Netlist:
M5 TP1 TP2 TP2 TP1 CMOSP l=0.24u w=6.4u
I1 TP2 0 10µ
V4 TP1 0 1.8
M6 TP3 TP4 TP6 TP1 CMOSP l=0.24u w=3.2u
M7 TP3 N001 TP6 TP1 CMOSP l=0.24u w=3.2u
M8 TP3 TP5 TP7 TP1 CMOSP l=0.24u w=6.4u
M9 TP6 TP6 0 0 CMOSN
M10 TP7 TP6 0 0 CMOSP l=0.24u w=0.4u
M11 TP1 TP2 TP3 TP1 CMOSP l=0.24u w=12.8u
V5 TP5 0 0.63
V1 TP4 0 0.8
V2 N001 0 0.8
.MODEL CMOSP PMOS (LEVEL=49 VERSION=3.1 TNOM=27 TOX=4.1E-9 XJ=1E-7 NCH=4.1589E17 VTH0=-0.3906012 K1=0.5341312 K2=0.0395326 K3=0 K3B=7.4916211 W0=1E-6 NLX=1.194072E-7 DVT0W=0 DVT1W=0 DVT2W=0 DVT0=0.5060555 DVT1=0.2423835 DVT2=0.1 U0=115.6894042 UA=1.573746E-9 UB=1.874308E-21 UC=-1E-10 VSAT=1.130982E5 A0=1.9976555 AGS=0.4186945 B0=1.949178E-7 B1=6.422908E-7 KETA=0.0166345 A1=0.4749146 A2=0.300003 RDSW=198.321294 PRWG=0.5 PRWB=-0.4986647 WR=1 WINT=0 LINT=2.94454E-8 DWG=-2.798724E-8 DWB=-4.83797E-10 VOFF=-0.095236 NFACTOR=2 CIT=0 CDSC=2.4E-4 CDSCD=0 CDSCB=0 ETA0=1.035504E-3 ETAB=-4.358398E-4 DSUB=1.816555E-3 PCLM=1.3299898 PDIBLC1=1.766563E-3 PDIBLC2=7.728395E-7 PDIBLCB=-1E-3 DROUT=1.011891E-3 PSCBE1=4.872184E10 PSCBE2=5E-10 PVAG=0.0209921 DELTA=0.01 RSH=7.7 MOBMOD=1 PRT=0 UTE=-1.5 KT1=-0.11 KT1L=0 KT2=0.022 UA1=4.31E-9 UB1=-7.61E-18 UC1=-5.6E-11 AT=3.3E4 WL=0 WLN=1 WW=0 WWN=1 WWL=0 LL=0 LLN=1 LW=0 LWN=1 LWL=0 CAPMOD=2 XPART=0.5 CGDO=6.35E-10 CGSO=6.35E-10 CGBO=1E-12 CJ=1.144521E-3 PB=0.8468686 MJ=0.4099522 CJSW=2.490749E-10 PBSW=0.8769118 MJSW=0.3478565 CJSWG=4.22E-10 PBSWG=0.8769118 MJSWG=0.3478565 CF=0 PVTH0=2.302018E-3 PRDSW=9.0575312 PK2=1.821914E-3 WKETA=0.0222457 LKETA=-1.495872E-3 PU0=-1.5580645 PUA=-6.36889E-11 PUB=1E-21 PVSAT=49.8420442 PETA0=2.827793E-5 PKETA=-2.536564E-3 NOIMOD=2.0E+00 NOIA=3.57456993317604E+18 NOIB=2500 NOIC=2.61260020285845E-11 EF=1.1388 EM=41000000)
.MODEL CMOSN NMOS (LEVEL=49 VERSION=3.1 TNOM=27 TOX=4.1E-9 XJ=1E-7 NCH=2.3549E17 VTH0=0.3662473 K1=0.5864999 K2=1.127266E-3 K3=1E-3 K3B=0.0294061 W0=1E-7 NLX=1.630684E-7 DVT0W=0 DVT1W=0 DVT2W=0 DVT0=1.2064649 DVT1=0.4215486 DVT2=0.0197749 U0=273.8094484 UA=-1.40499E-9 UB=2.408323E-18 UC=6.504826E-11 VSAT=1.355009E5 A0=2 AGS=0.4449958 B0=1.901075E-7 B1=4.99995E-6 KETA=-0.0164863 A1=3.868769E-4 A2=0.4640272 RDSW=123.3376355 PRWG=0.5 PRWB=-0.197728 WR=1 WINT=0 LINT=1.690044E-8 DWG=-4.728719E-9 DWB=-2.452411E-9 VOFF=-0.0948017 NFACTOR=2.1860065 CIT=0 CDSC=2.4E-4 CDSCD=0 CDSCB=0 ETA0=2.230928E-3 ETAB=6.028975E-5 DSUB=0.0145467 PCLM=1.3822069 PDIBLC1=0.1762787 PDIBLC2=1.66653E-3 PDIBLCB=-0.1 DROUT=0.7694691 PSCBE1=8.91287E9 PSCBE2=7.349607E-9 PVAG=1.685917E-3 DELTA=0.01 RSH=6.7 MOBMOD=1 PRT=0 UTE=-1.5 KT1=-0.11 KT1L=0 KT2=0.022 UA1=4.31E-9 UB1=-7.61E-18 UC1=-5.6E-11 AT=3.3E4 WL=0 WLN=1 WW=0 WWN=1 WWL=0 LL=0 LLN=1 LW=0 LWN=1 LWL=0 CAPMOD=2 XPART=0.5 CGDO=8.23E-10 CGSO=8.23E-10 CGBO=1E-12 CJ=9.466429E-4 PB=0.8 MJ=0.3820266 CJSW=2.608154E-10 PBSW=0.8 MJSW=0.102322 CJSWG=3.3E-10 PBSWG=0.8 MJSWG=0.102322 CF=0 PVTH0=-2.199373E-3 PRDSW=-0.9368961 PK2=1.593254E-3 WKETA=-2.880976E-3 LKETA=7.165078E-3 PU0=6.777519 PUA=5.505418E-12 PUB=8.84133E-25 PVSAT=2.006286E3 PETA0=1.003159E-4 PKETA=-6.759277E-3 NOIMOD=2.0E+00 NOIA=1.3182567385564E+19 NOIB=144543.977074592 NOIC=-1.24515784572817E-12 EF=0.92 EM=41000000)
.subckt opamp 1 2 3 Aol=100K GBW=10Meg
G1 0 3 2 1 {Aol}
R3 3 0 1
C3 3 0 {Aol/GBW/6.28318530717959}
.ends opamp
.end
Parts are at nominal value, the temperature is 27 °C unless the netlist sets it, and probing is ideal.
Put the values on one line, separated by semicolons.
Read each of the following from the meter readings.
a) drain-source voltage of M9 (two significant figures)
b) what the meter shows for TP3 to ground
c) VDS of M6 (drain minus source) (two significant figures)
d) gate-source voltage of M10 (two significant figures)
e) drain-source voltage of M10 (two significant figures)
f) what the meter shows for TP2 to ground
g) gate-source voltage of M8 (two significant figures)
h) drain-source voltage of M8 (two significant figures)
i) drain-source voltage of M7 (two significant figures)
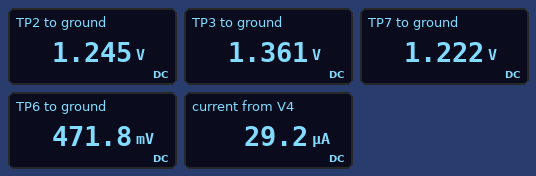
470 mV; 1.361 V; 890 mV; 470 mV; 1.2 V; 1.245 V; -590 mV; 140 mV; 890 mV
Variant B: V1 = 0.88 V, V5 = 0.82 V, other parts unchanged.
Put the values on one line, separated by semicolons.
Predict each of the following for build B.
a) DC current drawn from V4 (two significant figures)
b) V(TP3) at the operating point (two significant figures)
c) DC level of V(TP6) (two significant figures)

29 µA; 1.5 V; 670 mV
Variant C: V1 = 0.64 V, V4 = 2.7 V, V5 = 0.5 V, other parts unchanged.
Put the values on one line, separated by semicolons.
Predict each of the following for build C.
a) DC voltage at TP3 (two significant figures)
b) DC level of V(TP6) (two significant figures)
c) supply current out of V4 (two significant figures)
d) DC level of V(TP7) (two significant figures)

1.4 V; 490 mV; 32 µA; 1.3 V
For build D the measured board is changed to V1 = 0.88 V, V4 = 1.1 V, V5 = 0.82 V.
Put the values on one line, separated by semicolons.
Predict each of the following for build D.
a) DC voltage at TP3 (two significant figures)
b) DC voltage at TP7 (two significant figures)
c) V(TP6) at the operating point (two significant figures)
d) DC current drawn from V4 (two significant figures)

1.1 V; 530 mV; 300 mV; 10 µA
